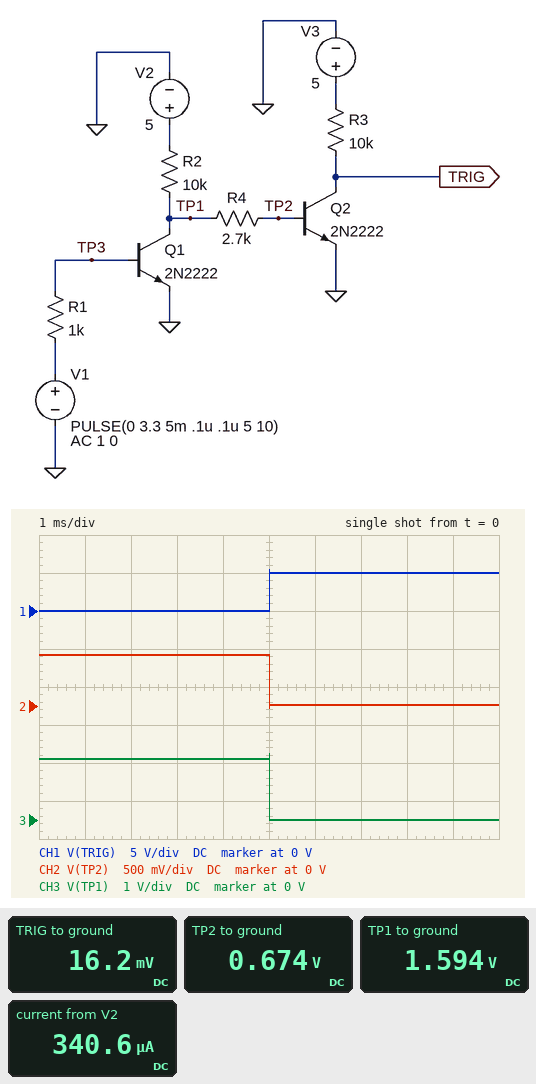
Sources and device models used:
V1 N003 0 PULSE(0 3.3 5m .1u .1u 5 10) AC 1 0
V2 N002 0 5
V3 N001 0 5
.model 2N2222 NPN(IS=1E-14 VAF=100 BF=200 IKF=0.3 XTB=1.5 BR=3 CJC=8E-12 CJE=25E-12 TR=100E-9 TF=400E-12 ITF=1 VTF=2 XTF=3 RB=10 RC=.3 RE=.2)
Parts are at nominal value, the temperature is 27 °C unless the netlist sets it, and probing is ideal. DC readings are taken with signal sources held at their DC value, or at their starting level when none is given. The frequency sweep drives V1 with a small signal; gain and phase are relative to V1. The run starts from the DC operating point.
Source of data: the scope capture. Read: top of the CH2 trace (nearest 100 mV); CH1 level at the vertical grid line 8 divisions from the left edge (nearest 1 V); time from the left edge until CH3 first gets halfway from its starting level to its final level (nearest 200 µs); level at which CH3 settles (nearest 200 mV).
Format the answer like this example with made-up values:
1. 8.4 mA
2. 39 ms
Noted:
1. 700 mV
2. 5 V
3. 5.0 ms
4. 0 V
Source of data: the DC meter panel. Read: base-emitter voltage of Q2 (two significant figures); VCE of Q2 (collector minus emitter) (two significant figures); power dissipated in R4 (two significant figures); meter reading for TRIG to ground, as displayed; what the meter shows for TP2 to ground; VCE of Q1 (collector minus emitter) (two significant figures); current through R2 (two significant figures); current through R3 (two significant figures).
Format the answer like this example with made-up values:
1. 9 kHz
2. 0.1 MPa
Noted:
1. 670 mV
2. 16 mV
3. 310 µW
4. 16.2 mV
5. 0.674 V
6. 1.6 V
7. 340 µA
8. 500 µA
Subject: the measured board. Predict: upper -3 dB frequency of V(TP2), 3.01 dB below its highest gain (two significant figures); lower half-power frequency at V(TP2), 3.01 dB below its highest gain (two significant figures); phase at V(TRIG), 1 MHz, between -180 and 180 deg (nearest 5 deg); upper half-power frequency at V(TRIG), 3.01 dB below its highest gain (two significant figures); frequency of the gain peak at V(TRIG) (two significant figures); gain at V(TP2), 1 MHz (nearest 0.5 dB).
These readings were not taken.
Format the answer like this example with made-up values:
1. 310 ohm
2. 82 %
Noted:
1. 25 MHz
2. 2.9 MHz
3. 140 deg
4. 26 MHz
5. 9.1 MHz
6. -60.0 dB
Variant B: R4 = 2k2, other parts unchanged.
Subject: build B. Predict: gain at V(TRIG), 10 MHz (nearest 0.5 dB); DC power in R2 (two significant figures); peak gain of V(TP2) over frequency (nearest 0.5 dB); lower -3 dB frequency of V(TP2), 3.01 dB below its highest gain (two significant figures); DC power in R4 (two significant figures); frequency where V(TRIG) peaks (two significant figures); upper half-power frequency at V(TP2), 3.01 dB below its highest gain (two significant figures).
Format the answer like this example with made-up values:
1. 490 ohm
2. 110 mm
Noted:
1. -56.0 dB
2. 1.3 mW
3. -51.5 dB
4. 3.0 MHz
5. 280 µW
6. 9.8 MHz
7. 28 MHz
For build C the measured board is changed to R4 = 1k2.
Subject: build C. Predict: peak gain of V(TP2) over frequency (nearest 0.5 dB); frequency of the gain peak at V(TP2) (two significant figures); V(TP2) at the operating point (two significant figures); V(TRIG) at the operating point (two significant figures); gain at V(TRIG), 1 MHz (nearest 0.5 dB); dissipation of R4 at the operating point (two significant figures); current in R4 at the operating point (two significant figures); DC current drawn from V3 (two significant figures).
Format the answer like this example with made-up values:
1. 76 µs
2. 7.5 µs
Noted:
1. -50.0 dB
2. 12 MHz
3. 680 mV
4. 15 mV
5. -67.0 dB
6. 180 µW
7. 390 µA
8. 500 µA
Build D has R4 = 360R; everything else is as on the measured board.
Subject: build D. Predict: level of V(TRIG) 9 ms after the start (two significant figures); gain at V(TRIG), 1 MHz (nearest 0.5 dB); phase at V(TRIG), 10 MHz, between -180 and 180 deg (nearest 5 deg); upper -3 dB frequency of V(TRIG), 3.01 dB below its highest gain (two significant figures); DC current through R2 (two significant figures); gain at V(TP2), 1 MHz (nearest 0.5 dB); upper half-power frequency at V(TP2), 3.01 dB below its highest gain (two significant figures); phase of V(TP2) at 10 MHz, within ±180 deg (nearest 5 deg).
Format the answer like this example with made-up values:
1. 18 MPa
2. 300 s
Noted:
1. 5.0 V
2. -66.5 dB
3. 25 deg
4. 82 MHz
5. 420 µA
6. -58.0 dB
7. 84 MHz
8. 15 deg
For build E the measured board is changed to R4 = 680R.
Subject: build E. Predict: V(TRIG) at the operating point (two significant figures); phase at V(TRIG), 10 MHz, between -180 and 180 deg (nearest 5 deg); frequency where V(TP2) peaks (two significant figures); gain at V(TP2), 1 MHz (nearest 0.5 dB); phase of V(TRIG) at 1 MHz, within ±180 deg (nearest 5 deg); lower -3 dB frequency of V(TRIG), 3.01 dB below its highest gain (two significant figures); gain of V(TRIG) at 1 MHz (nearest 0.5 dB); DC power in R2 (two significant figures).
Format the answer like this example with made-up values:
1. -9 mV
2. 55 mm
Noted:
1. 15 mV
2. 20 deg
3. 15 MHz
4. -58.5 dB
5. 140 deg
6. 4.1 MHz
7. -66.5 dB
8. 1.6 mW
